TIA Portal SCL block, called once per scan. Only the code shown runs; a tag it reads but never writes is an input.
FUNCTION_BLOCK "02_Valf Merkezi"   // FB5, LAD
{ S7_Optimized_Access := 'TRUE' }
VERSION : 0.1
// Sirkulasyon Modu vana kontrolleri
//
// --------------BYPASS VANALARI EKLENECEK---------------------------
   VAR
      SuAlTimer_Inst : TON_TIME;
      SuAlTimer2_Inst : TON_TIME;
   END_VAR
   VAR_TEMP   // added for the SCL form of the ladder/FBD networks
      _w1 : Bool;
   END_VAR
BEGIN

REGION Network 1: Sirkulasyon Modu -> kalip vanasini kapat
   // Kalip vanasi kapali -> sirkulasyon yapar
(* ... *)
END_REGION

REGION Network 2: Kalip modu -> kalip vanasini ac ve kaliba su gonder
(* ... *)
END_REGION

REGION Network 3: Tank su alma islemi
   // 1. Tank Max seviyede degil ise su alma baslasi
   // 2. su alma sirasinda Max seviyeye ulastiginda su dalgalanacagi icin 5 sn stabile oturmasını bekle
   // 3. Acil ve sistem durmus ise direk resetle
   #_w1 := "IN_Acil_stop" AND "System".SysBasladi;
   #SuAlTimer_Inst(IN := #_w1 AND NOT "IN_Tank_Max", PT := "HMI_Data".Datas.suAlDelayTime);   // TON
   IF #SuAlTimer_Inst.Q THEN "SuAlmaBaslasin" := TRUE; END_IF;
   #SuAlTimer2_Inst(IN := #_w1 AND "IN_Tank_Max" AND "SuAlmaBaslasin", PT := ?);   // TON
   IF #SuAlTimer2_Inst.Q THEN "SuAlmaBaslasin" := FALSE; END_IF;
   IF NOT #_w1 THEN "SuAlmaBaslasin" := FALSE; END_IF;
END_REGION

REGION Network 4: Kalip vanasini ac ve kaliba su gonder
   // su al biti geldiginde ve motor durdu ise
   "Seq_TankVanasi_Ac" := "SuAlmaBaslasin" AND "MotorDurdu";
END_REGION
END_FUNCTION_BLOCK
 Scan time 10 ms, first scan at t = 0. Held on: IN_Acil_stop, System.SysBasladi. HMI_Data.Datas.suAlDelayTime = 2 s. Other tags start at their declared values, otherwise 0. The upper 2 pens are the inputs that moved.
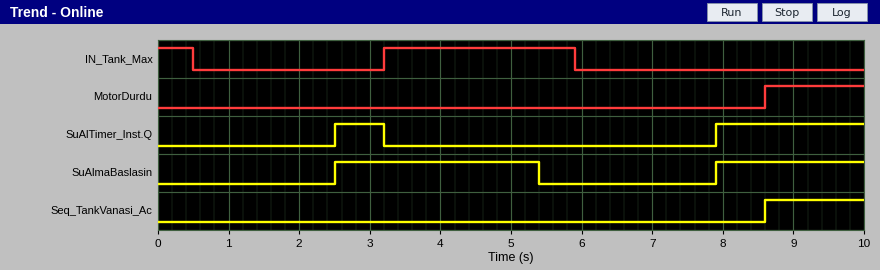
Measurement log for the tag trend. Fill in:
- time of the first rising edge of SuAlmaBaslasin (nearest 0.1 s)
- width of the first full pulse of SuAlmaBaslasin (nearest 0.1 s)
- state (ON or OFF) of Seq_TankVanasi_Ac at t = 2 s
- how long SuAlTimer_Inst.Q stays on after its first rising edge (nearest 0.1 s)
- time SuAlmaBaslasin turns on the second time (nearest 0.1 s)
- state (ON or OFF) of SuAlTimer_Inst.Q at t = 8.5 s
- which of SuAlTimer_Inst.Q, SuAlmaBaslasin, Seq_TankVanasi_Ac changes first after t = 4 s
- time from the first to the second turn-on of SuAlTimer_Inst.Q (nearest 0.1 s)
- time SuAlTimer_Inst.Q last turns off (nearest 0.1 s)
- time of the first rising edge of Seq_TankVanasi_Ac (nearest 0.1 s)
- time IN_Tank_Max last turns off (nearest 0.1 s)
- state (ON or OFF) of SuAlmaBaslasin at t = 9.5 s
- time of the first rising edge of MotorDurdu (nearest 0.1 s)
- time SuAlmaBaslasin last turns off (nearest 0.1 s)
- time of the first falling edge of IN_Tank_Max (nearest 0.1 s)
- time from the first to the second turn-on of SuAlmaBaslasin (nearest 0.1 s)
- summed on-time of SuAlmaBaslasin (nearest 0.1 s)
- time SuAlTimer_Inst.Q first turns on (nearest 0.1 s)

2.5 s
2.9 s
OFF
0.7 s
7.9 s
ON
SuAlmaBaslasin
5.4 s
3.2 s
8.6 s
5.9 s
ON
8.6 s
5.4 s
0.5 s
5.4 s
5.0 s
2.5 s
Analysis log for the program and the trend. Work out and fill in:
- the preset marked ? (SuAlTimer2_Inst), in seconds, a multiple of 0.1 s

2.2 s
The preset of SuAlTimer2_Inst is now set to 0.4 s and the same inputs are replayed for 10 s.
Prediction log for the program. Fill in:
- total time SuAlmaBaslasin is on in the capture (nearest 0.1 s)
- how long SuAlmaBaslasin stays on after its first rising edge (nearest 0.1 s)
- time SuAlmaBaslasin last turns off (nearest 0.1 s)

3.2 s
1.1 s
3.6 s
